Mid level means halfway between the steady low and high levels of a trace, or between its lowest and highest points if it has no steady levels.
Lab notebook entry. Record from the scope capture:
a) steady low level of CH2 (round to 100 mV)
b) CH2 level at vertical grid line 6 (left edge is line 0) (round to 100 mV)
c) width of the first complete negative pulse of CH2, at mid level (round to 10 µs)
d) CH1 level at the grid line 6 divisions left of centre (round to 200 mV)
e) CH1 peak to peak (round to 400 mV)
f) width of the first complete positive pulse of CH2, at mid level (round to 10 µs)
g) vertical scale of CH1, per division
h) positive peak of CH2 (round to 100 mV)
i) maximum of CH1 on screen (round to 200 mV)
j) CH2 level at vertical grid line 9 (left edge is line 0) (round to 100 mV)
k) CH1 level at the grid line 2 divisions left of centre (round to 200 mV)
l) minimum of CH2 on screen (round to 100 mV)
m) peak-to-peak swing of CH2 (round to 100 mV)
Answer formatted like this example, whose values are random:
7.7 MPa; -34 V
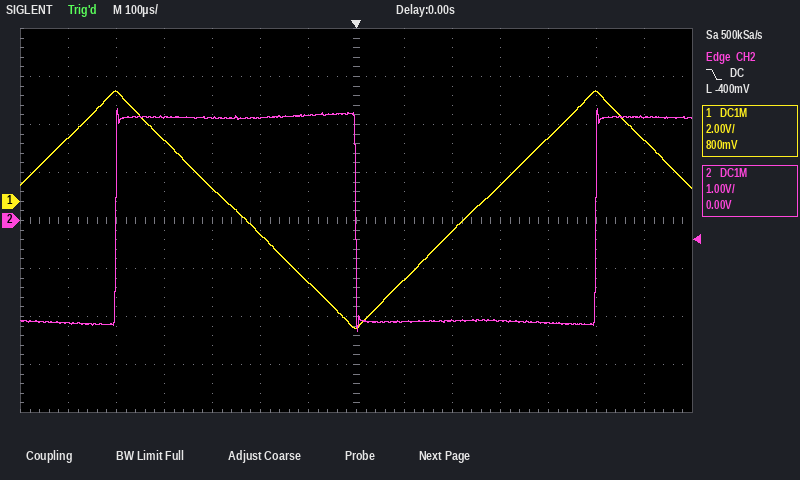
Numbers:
-2.1 V; 2.2 V; 500 µs; 2.6 V; 10.0 V; 500 µs; 2 V; 2.3 V; 4.6 V; -2.1 V; -1.4 V; -2.3 V; 4.6 V
